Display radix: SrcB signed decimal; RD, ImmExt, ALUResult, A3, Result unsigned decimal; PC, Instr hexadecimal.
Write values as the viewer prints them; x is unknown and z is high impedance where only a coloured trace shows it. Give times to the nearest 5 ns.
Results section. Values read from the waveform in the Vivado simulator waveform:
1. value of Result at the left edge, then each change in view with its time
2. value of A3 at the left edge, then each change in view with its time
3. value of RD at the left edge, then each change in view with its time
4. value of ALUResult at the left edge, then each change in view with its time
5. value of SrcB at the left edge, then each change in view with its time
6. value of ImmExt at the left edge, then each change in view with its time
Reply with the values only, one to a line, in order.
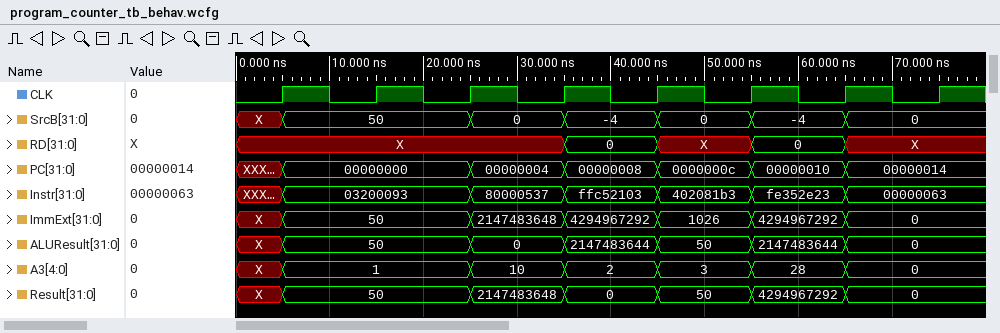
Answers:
X, 50 at 5 ns, 2147483648 at 25 ns, 0 at 35 ns, 50 at 45 ns, 4294967292 at 55 ns, 0 at 65 ns
X, 1 at 5 ns, 10 at 25 ns, 2 at 35 ns, 3 at 45 ns, 28 at 55 ns, 0 at 65 ns
X, 0 at 35 ns, X at 45 ns, 0 at 55 ns, X at 65 ns
X, 50 at 5 ns, 0 at 25 ns, 2147483644 at 35 ns, 50 at 45 ns, 2147483644 at 55 ns, 0 at 65 ns
X, 50 at 5 ns, 0 at 25 ns, -4 at 35 ns, 0 at 45 ns, -4 at 55 ns, 0 at 65 ns
X, 50 at 5 ns, 2147483648 at 25 ns, 4294967292 at 35 ns, 1026 at 45 ns, 4294967292 at 55 ns, 0 at 65 ns
